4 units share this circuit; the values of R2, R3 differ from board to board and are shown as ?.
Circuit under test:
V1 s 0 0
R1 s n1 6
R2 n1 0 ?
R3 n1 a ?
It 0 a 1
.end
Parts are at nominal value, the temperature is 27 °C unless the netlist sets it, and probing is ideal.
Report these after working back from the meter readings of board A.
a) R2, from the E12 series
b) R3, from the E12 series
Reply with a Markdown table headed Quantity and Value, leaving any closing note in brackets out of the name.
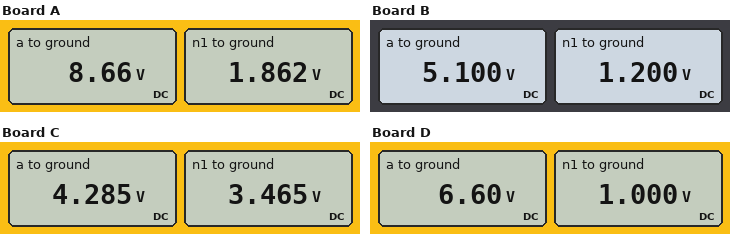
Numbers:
| Quantity | Value |
|---|---|
| R2, from the E12 series | 2.7 Ω |
| R3, from the E12 series | 6.8 Ω |
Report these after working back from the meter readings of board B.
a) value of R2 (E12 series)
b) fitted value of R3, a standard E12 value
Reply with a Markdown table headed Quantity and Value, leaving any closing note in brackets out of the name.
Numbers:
| Quantity | Value |
|---|---|
| value of R2 | 1.5 Ω |
| fitted value of R3, a standard E12 value | 3.9 Ω |
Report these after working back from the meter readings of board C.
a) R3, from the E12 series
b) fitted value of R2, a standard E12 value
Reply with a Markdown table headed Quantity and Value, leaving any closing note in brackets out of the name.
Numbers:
| Quantity | Value |
|---|---|
| R3, from the E12 series | 0.82 Ω |
| fitted value of R2, a standard E12 value | 8.2 Ω |
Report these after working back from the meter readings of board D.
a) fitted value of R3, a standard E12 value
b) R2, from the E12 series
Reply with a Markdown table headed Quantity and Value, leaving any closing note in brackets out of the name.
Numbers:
| Quantity | Value |
|---|---|
| fitted value of R3, a standard E12 value | 5.6 Ω |
| R2, from the E12 series | 1.2 Ω |
